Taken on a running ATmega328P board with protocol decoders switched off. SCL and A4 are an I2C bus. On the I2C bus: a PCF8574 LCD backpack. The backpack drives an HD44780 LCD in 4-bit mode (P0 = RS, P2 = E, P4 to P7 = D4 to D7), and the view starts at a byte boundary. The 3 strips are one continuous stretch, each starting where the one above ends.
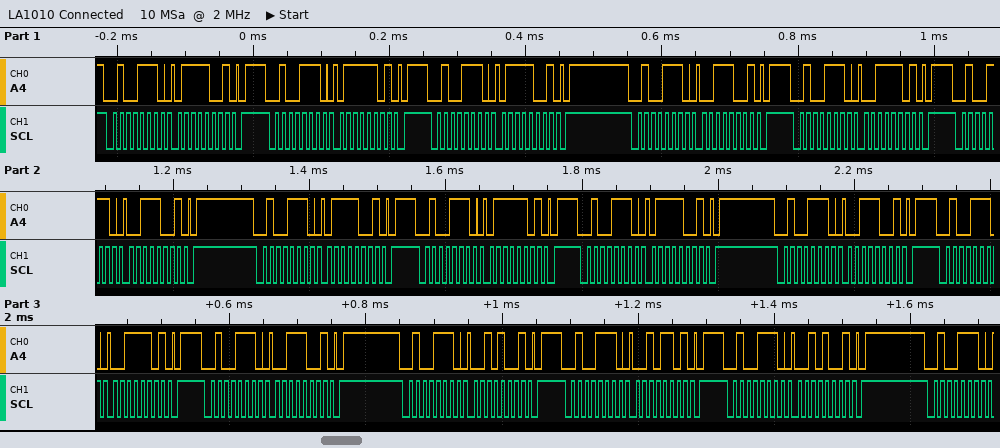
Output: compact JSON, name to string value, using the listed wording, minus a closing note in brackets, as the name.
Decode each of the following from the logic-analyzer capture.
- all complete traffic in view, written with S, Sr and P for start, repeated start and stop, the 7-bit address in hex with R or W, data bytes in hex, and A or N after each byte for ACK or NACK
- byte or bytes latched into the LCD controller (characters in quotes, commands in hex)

{"all complete traffic in view, written with S, Sr and P for start, repeated start and stop, the 7-bit address in hex with R or W, data bytes in hex, and A or N after each byte for ACK or NACK": "S 27W A 79 A P S 27W A 7D A P S 27W A 79 A P S 27W A 39 A P S 27W A 3D A P S 27W A 39 A P S 27W A 79 A P S 27W A 7D A P S 27W A 79 A P S 27W A 39 A P S 27W A 3D A P S 27W A 39 A P S 27W A 29 A P S 27W A 2D A P S 27W A 29 A P S 27W A", "byte or bytes latched into the LCD controller": "'s' 's'"}
